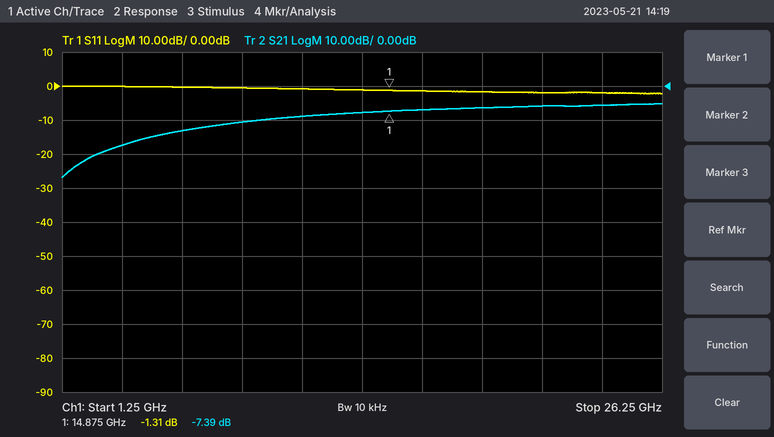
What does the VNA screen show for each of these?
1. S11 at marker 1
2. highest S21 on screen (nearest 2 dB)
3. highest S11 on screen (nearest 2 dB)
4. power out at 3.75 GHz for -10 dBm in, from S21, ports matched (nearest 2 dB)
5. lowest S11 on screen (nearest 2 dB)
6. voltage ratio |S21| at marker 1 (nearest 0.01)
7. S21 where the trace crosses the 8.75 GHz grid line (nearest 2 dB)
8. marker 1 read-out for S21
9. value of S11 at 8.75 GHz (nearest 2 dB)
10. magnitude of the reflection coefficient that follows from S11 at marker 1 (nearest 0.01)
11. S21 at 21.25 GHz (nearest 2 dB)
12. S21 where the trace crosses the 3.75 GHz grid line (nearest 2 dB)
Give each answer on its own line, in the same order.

-1.31 dB
-6 dB
0 dB
-28 dBm
-2 dB
0.43
-10 dB
-7.39 dB
0 dB
0.86
-6 dB
-18 dB
